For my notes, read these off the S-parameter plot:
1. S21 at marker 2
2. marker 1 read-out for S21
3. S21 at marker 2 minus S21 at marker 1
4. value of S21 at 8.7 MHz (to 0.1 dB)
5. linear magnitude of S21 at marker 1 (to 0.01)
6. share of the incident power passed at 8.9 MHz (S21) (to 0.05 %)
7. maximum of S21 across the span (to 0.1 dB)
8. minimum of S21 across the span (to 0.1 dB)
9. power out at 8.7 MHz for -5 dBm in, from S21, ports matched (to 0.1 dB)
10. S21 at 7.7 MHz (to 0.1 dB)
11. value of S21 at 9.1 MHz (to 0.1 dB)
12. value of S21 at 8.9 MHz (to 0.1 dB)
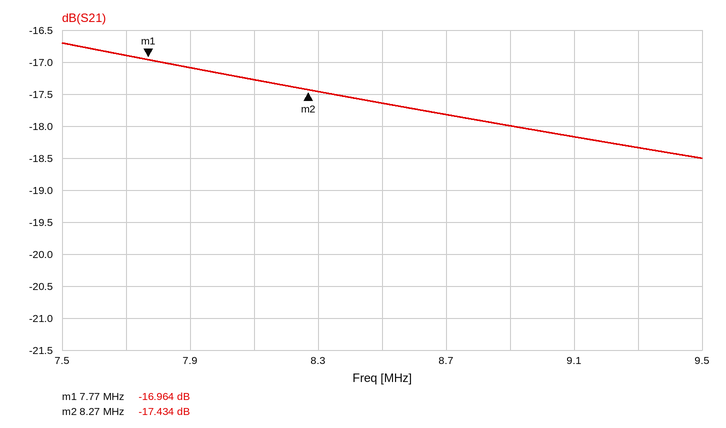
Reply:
-17.434 dB
-16.964 dB
-0.470 dB
-17.8 dB
0.14
1.60 %
-16.7 dB
-18.5 dB
-22.8 dBm
-16.9 dB
-18.2 dB
-18.0 dB
